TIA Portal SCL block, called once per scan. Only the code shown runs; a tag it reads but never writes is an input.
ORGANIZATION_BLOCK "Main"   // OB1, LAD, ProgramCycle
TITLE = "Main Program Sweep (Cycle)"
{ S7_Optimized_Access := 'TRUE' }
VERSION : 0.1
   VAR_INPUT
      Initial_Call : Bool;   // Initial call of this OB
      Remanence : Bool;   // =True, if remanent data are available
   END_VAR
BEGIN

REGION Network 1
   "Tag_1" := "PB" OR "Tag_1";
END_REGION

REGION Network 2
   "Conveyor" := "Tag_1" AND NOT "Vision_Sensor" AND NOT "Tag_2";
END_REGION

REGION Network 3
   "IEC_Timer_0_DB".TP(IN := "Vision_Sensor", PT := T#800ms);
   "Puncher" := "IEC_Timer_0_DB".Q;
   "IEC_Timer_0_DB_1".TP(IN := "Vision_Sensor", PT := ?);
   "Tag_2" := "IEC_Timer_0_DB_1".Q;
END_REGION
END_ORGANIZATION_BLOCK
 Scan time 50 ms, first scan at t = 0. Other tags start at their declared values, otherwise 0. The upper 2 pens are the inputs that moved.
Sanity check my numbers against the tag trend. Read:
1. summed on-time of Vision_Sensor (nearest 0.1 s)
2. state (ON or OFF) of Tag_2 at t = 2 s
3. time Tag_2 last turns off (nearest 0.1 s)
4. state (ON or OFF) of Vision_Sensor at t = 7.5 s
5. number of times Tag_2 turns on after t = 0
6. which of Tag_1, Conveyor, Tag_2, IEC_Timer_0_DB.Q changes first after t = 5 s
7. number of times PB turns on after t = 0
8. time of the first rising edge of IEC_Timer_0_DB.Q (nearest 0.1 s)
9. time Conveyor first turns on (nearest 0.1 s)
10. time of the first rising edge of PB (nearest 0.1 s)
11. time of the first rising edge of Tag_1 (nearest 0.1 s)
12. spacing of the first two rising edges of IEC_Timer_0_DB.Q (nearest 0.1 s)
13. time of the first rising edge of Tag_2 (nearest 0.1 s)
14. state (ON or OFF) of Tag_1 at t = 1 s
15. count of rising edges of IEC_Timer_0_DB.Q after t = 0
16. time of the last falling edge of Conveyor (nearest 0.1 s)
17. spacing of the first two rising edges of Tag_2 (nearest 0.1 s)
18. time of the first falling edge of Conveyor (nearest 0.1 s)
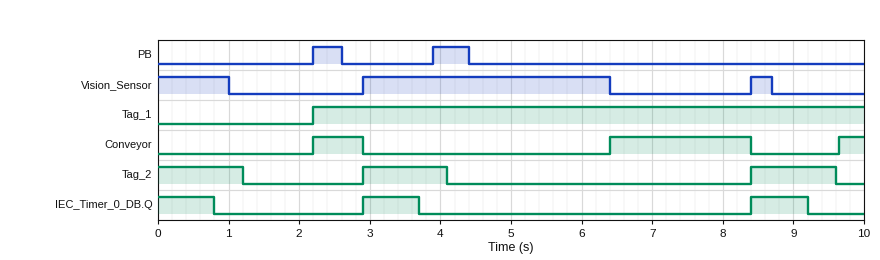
4.8 s
OFF
9.6 s
OFF
2
Conveyor
2
2.9 s
2.2 s
2.2 s
2.2 s
5.5 s
2.9 s
OFF
2
8.4 s
5.5 s
2.9 s
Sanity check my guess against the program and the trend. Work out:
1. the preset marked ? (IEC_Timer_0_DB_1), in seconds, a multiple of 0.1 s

1.2 s
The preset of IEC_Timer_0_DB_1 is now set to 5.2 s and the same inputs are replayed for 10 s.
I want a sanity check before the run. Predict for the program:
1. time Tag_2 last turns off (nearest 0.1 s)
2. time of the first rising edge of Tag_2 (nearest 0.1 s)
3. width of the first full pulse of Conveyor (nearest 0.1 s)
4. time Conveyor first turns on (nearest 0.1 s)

5.2 s
8.4 s
2.0 s
6.4 s
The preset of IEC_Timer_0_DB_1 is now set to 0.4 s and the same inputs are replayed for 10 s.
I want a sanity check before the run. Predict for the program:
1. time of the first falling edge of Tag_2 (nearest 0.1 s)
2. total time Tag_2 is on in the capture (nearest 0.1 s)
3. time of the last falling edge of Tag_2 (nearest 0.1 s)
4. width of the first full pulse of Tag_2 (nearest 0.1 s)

0.4 s
1.2 s
8.8 s
0.4 s
